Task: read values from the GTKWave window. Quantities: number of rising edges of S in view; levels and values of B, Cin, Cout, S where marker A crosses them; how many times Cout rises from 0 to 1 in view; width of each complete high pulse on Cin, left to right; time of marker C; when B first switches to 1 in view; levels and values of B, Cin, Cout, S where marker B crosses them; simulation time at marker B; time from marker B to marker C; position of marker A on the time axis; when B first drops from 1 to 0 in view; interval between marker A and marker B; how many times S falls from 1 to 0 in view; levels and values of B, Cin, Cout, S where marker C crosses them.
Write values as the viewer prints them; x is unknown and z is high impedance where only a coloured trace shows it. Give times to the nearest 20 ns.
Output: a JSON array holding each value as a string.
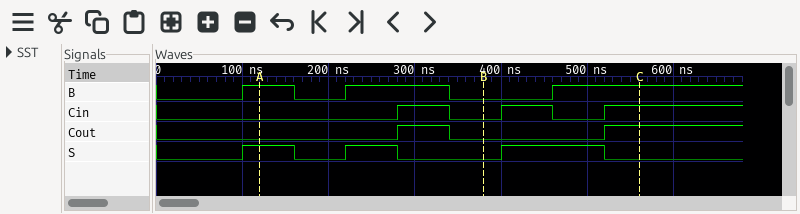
["3", "B=1, Cin=0, Cout=0, S=1", "2", "60 ns, 60 ns", "560 ns", "100 ns", "B=0, Cin=0, Cout=0, S=0", "380 ns", "180 ns", "120 ns", "160 ns", "260 ns", "3", "B=1, Cin=1, Cout=1, S=0"]
